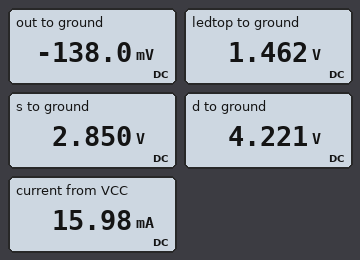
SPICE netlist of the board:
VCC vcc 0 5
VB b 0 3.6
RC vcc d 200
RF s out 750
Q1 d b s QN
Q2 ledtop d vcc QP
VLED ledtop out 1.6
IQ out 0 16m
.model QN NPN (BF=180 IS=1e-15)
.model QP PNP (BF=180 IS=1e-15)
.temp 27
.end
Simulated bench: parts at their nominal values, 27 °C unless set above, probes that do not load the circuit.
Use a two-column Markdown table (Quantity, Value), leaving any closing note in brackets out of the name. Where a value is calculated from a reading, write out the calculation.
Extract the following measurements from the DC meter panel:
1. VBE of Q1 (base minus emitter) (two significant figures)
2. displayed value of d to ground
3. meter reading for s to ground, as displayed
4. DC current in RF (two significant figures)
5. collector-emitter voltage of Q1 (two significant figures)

| Quantity | Value |
|---|---|
| VBE of Q1 (base minus emitter) | 3.6 V - 2.85 V = 750 mV |
| displayed value of d to ground | 4.221 V |
| meter reading for s to ground, as displayed | 2.850 V |
| DC current in RF | (2.85 V - (-138 mV)) / 750 Ω = 4.0 mA |
| collector-emitter voltage of Q1 | 4.221 V - 2.85 V = 1.4 V |
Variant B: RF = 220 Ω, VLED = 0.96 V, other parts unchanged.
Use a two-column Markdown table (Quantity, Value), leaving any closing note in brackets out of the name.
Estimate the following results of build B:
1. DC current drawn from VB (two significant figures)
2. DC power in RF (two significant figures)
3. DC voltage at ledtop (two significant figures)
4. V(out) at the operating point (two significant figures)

| Quantity | Value |
|---|---|
| DC current drawn from VB | 22 µA |
| DC power in RF | 3.5 mW |
| DC voltage at ledtop | 2.9 V |
| V(out) at the operating point | 2.0 V |
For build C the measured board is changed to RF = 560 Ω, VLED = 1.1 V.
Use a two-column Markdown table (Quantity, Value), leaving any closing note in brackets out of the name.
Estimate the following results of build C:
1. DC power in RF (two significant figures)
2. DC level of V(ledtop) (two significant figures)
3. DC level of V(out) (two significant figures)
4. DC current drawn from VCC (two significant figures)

| Quantity | Value |
|---|---|
| DC power in RF | 8.9 mW |
| DC level of V(ledtop) | 1.7 V |
| DC level of V(out) | 620 mV |
| DC current drawn from VCC | 16 mA |
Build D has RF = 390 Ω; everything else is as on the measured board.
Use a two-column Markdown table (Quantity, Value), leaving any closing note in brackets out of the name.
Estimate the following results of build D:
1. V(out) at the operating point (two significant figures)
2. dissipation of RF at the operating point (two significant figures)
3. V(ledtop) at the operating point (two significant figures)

| Quantity | Value |
|---|---|
| V(out) at the operating point | 1.3 V |
| dissipation of RF at the operating point | 6.2 mW |
| V(ledtop) at the operating point | 2.9 V |
